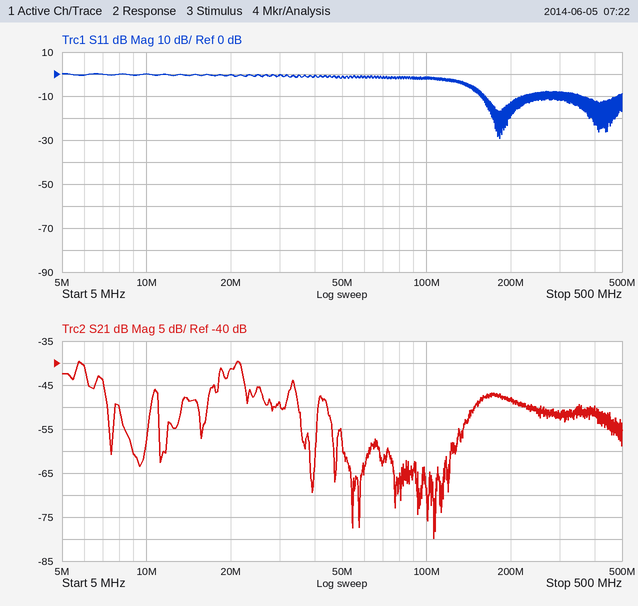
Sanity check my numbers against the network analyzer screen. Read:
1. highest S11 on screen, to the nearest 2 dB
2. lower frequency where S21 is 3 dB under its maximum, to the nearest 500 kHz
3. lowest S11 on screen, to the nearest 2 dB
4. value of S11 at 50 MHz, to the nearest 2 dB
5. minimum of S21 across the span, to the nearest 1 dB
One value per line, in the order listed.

0 dB
5.5 MHz
-30 dB
-2 dB
-80 dB
